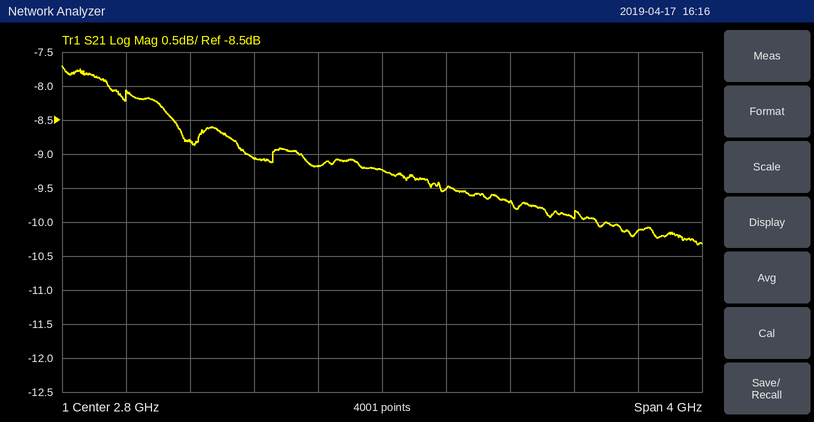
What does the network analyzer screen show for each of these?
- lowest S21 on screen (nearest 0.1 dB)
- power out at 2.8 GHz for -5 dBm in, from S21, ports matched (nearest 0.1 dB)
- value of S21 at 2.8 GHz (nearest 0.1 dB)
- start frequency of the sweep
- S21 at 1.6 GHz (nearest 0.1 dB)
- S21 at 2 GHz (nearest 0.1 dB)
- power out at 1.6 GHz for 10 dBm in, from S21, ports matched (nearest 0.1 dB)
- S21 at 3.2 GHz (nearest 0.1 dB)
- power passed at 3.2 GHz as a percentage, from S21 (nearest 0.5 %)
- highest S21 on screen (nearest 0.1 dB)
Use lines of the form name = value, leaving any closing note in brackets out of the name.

lowest S21 on screen = -10.3 dB
power out at 2.8 GHz for -5 dBm in, from S21, ports matched = -14.2 dBm
value of S21 at 2.8 GHz = -9.2 dB
start frequency of the sweep = 800 MHz
S21 at 1.6 GHz = -8.8 dB
S21 at 2 GHz = -9.1 dB
power out at 1.6 GHz for 10 dBm in, from S21, ports matched = 1.2 dBm
S21 at 3.2 GHz = -9.5 dB
power passed at 3.2 GHz as a percentage, from S21 = 11.0 %
highest S21 on screen = -7.7 dB
